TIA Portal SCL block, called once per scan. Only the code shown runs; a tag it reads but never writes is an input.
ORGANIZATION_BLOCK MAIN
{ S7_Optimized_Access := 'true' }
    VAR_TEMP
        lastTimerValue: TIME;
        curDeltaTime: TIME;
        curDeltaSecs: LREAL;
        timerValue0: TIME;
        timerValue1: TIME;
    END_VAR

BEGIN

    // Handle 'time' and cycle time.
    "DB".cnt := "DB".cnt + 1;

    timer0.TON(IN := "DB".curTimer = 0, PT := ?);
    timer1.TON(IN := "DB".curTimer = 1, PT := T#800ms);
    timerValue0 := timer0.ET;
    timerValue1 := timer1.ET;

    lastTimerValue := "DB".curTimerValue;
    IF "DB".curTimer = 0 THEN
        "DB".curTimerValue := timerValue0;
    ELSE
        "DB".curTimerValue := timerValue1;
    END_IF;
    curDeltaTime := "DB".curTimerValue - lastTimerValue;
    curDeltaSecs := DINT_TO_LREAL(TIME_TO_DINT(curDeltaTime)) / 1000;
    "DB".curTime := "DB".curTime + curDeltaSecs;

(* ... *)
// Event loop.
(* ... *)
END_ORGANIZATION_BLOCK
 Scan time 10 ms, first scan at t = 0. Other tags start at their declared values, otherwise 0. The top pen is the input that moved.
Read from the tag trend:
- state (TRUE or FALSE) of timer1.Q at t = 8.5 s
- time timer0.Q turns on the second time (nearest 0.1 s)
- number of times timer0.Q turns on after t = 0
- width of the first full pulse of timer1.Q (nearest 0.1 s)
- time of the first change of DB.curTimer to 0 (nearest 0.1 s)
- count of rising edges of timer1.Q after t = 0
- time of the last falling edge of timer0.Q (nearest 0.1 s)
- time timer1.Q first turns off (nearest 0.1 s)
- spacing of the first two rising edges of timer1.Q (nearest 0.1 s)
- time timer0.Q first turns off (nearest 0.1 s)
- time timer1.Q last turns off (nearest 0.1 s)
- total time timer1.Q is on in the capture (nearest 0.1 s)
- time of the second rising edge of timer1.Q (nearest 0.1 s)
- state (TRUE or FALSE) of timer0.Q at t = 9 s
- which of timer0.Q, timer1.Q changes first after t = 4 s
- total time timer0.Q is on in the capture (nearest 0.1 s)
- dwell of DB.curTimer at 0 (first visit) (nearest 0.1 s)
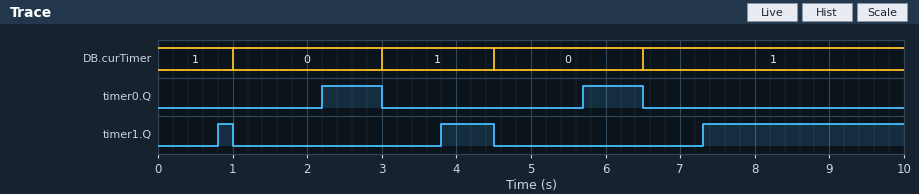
TRUE
5.7 s
2
0.2 s
1.0 s
3
6.5 s
1.0 s
3.0 s
3.0 s
4.5 s
3.6 s
3.8 s
FALSE
timer1.Q
1.6 s
2.0 s
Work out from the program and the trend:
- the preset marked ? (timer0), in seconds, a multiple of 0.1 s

1.2 s
